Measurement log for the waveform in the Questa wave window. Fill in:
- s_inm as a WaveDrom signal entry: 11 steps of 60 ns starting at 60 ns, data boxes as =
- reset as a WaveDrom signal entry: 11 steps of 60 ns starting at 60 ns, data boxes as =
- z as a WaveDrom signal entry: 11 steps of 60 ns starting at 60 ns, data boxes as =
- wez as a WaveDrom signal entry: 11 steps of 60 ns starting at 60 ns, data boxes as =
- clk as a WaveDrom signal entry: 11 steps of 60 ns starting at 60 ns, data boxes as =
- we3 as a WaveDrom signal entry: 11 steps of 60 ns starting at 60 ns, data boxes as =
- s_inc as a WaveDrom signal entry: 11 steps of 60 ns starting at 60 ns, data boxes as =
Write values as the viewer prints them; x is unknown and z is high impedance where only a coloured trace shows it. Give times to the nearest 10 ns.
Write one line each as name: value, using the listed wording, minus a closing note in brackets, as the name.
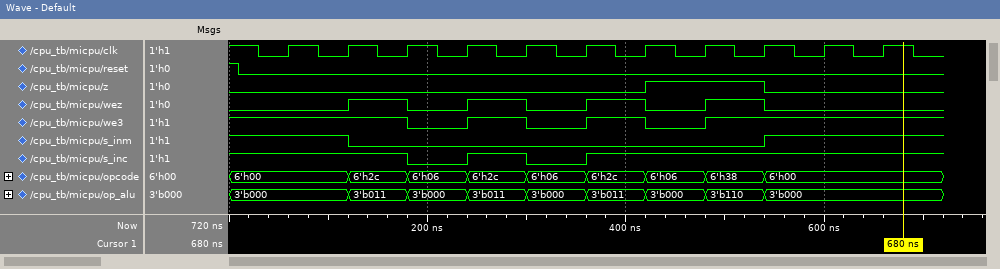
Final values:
s_inm as a WaveDrom signal entry: 11 steps of 60 ns starting at 60 ns, data boxes as =: {name: 's_inm', wave: '10......1..'}
reset as a WaveDrom signal entry: 11 steps of 60 ns starting at 60 ns, data boxes as =: {name: 'reset', wave: '0..........'}
z as a WaveDrom signal entry: 11 steps of 60 ns starting at 60 ns, data boxes as =: {name: 'z', wave: '0.....1.0..'}
wez as a WaveDrom signal entry: 11 steps of 60 ns starting at 60 ns, data boxes as =: {name: 'wez', wave: '010101010..'}
clk as a WaveDrom signal entry: 11 steps of 60 ns starting at 60 ns, data boxes as =: {name: 'clk', wave: 'p..........'}
we3 as a WaveDrom signal entry: 11 steps of 60 ns starting at 60 ns, data boxes as =: {name: 'we3', wave: '1.010101...'}
s_inc as a WaveDrom signal entry: 11 steps of 60 ns starting at 60 ns, data boxes as =: {name: 's_inc', wave: '1.0101.....'}
